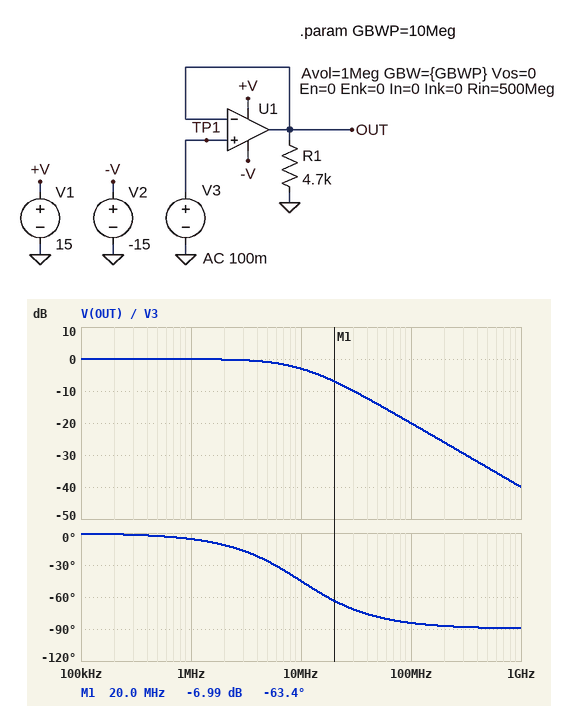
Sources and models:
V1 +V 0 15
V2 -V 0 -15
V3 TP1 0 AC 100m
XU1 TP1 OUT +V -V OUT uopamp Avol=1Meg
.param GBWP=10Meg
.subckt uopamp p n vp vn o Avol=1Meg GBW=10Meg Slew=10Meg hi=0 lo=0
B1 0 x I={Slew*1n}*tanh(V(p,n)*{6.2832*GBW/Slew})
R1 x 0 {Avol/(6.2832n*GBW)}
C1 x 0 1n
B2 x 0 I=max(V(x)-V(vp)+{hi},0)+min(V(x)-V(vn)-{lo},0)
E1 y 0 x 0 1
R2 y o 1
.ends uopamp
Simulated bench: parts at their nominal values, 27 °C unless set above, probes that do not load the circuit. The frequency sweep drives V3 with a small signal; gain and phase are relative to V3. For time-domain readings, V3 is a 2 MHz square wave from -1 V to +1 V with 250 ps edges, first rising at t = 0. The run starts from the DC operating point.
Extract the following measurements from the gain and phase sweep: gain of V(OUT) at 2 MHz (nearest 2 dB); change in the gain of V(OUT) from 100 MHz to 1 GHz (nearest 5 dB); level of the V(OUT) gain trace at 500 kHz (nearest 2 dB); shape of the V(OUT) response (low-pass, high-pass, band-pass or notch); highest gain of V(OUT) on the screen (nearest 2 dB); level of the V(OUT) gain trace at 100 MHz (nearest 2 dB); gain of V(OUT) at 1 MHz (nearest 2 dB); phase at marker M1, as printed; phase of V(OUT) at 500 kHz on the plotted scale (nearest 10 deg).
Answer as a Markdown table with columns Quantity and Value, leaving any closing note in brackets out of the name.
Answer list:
| Quantity | Value |
|---|---|
| gain of V(OUT) at 2 MHz | 0 dB |
| change in the gain of V(OUT) from 100 MHz to 1 GHz | -20 dB |
| level of the V(OUT) gain trace at 500 kHz | 0 dB |
| shape of the V(OUT) response | low-pass |
| highest gain of V(OUT) on the screen | 0 dB |
| level of the V(OUT) gain trace at 100 MHz | -20 dB |
| gain of V(OUT) at 1 MHz | 0 dB |
| phase at marker M1, as printed | -63.4 deg |
| phase of V(OUT) at 500 kHz on the plotted scale | 0 deg |
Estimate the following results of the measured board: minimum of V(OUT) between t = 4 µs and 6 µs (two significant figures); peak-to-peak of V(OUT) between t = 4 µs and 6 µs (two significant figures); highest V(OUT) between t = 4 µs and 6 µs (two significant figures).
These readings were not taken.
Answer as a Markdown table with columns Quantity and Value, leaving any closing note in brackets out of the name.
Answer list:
| Quantity | Value |
|---|---|
| minimum of V(OUT) between t = 4 µs and 6 µs | -1.0 V |
| peak-to-peak of V(OUT) between t = 4 µs and 6 µs | 2.0 V |
| highest V(OUT) between t = 4 µs and 6 µs | 1.0 V |
